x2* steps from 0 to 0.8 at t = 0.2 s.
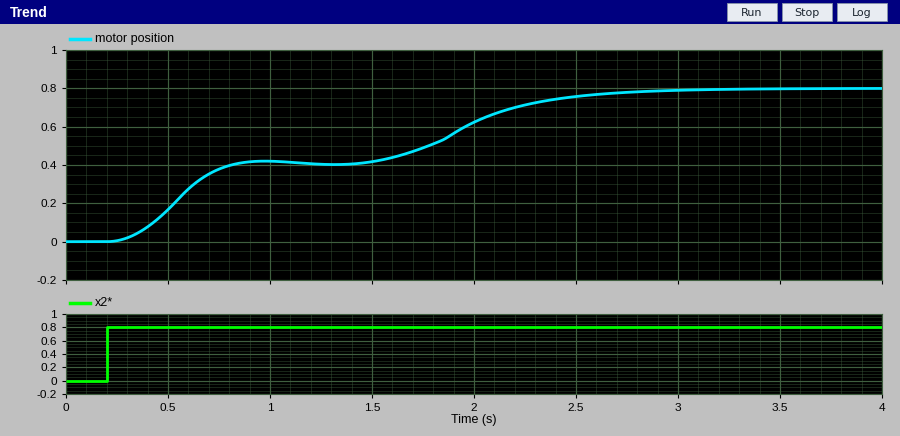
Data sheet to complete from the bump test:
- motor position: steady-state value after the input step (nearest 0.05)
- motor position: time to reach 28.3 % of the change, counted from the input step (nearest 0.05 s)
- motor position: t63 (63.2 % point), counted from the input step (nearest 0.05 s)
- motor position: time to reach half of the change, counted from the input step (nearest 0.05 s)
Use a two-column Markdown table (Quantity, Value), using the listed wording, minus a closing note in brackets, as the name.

| Quantity | Value |
|---|---|
| motor position: steady-state value after the input step | 0.80 |
| motor position: time to reach 28.3 % of the change, counted from the input step | 0.35 s |
| motor position: t63 (63.2 % point), counted from the input step | 1.60 s |
| motor position: time to reach half of the change, counted from the input step | 0.60 s |
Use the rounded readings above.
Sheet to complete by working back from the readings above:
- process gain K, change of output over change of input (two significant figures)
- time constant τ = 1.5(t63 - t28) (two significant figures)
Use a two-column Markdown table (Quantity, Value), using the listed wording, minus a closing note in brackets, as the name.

| Quantity | Value |
|---|---|
| process gain K, change of output over change of input | 1.0 |
| time constant τ = 1.5(t63 - t28) | 1.9 s |
